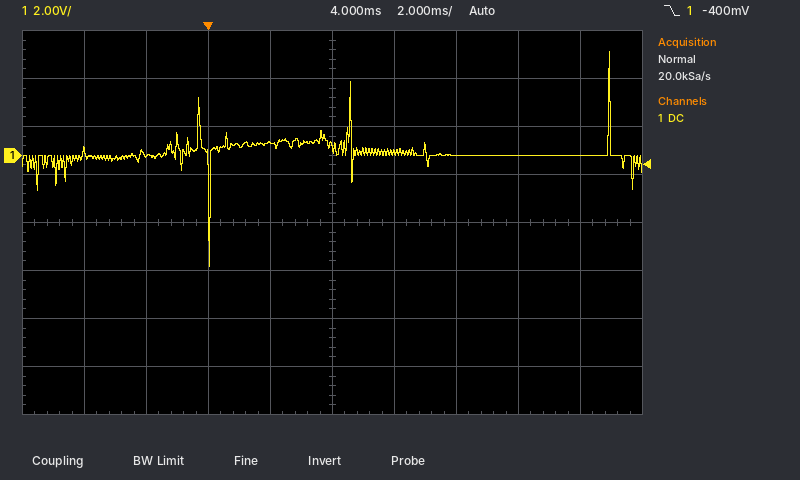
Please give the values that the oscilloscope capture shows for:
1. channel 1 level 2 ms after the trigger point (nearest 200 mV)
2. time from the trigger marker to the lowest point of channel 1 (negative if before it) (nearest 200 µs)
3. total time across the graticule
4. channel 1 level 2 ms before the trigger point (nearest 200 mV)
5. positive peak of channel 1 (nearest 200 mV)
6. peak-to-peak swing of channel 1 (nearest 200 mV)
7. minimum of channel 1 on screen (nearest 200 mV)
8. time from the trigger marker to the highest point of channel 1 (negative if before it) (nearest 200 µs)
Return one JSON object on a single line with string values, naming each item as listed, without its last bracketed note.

{"channel 1 level 2 ms after the trigger point": "600 mV", "time from the trigger marker to the lowest point of channel 1 (negative if before it)": "0.0 ms", "total time across the graticule": "20 ms", "channel 1 level 2 ms before the trigger point": "0.0 V", "positive peak of channel 1": "4.4 V", "peak-to-peak swing of channel 1": "9.0 V", "minimum of channel 1 on screen": "-4.6 V", "time from the trigger marker to the highest point of channel 1 (negative if before it)": "+13.0 ms"}
